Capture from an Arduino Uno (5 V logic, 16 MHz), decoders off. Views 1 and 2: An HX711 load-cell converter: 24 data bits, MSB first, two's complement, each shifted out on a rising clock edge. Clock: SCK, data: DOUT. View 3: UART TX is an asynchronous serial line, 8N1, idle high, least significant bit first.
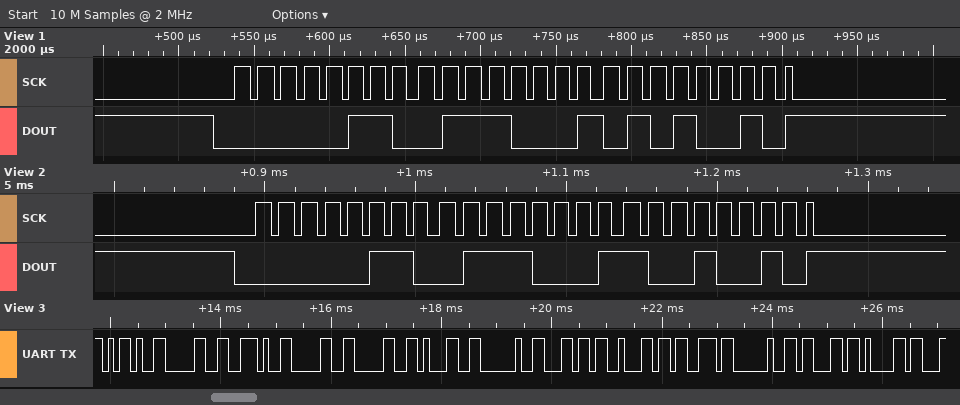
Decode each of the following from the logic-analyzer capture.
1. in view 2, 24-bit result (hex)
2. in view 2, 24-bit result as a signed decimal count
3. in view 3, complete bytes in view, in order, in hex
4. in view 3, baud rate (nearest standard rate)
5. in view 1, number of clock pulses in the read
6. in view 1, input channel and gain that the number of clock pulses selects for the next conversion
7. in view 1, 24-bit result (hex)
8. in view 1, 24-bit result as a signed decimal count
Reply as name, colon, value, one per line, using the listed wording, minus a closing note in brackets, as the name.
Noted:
in view 2, 24-bit result: 0x067192
in view 2, 24-bit result as a signed decimal count: 422290
in view 3, complete bytes in view, in order, in hex: 2D 30 2E 30 30 31 20 6C 62 73 20 63 61
in view 3, baud rate: 9600 baud
in view 1, number of clock pulses in the read: 25
in view 1, input channel and gain that the number of clock pulses selects for the next conversion: channel A, gain 128
in view 1, 24-bit result: 0x067152
in view 1, 24-bit result as a signed decimal count: 422226
